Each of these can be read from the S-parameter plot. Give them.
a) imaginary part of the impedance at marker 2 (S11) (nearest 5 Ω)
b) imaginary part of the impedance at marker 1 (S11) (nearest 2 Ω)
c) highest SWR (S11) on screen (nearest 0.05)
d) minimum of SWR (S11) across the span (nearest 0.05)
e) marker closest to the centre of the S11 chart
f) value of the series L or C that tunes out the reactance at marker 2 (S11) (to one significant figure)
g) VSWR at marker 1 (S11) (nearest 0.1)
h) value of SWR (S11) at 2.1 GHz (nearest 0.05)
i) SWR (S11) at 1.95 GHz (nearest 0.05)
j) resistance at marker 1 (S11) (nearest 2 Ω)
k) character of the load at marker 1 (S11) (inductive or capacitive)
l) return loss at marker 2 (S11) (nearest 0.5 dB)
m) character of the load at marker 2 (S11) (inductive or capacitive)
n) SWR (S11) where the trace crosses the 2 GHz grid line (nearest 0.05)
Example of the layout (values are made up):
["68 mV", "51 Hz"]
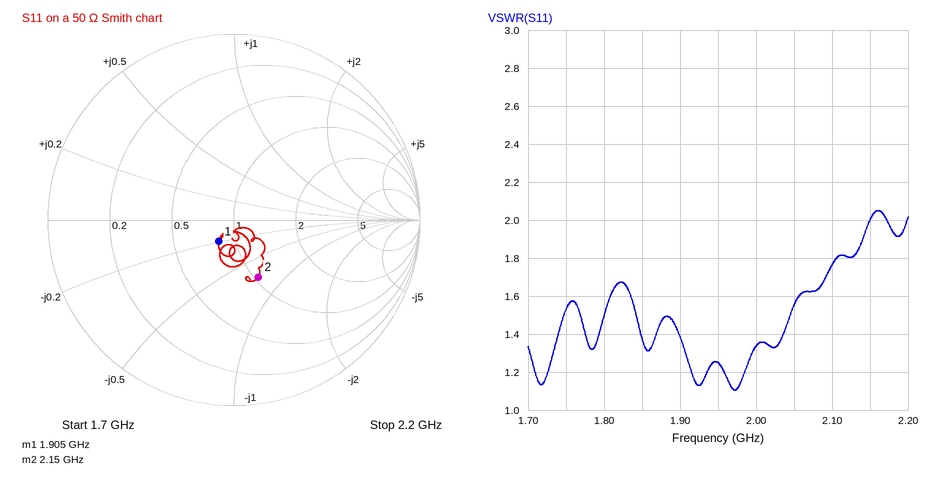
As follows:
["-35 Ω", "-10 Ω", "2.05", "1.10", "marker 1", "3 nH", "1.3", "1.75", "1.25", "42 Ω", "capacitive", "9.5 dB", "capacitive", "1.35"]
